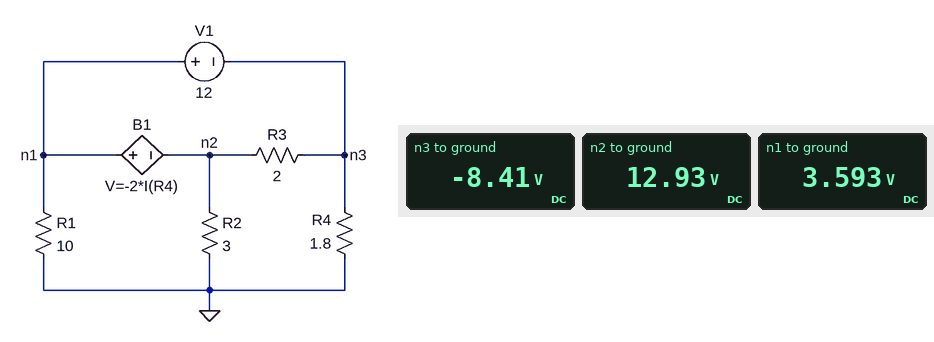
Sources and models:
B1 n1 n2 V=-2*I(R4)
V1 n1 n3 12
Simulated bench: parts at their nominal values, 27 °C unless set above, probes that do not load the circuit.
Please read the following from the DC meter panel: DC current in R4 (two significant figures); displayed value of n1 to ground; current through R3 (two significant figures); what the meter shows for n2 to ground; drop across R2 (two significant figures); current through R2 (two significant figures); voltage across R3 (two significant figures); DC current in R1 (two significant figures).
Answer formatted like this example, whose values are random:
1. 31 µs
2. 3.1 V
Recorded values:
1. 4.7 A
2. 3.593 V
3. 11 A
4. 12.93 V
5. 13 V
6. 4.3 A
7. 21 V
8. 360 mA
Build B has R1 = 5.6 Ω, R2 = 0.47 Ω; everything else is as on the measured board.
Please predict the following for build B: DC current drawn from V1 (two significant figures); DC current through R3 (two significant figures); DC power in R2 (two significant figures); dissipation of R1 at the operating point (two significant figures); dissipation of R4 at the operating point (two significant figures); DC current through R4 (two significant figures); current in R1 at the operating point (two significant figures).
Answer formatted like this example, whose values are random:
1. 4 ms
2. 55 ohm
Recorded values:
1. 68 A
2. 37 A
3. 700 W
4. 340 W
5. 1.7 kW
6. 31 A
7. 7.8 A
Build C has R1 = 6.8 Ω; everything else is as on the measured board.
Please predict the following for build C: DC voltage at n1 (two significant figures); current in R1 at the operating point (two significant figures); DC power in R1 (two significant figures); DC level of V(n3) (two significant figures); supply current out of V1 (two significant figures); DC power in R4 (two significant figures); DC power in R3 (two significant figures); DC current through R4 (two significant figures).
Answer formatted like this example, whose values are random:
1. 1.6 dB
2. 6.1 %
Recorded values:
1. 3.3 V
2. 490 mA
3. 1.6 W
4. -8.7 V
5. 16 A
6. 42 W
7. 230 W
8. 4.8 A
